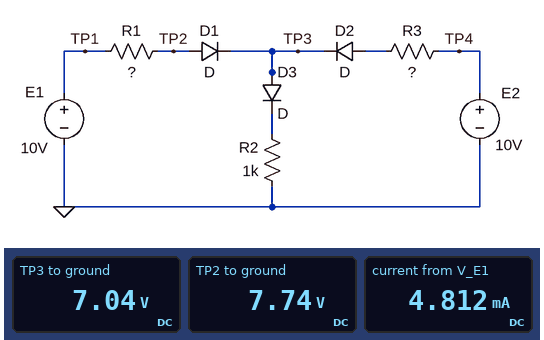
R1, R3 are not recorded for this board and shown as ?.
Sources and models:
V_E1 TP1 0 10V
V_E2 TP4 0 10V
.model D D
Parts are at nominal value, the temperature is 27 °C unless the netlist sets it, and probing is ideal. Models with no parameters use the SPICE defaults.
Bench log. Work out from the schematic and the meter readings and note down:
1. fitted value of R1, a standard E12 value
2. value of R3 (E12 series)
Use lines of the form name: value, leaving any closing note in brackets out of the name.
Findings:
fitted value of R1, a standard E12 value: 470 Ω
value of R3: 1.5 kΩ
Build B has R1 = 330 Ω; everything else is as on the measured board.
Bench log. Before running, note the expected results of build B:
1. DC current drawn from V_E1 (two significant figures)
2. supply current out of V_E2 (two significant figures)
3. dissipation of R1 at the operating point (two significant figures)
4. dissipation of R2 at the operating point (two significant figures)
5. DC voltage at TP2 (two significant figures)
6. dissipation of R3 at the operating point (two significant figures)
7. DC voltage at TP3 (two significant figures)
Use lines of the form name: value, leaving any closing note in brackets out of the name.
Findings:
DC current drawn from V_E1: 5.5 mA
supply current out of V_E2: 1.2 mA
dissipation of R1 at the operating point: 10 mW
dissipation of R2 at the operating point: 46 mW
DC voltage at TP2: 8.2 V
dissipation of R3 at the operating point: 2.3 mW
DC voltage at TP3: 7.5 V
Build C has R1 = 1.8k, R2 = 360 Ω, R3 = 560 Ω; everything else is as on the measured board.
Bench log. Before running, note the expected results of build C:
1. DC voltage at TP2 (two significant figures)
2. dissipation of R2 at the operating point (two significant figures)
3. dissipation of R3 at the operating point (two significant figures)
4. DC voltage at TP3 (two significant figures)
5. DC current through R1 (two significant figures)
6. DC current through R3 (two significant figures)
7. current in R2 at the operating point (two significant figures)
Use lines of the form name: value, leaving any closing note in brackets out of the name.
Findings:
DC voltage at TP2: 5.3 V
dissipation of R2 at the operating point: 43 mW
dissipation of R3 at the operating point: 39 mW
DC voltage at TP3: 4.6 V
DC current through R1: 2.6 mA
DC current through R3: 8.3 mA
current in R2 at the operating point: 11 mA
